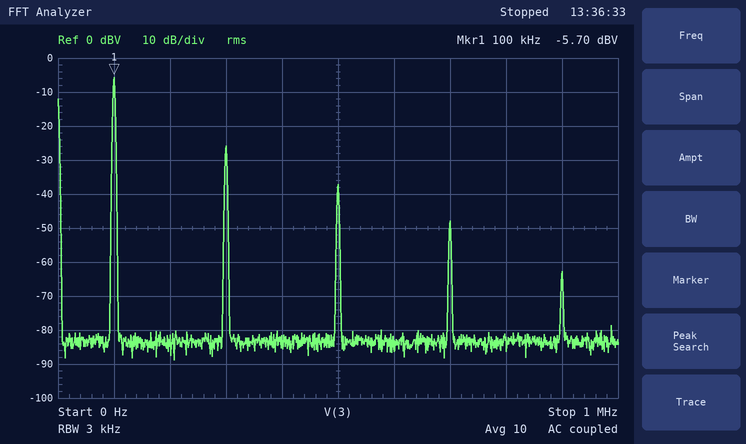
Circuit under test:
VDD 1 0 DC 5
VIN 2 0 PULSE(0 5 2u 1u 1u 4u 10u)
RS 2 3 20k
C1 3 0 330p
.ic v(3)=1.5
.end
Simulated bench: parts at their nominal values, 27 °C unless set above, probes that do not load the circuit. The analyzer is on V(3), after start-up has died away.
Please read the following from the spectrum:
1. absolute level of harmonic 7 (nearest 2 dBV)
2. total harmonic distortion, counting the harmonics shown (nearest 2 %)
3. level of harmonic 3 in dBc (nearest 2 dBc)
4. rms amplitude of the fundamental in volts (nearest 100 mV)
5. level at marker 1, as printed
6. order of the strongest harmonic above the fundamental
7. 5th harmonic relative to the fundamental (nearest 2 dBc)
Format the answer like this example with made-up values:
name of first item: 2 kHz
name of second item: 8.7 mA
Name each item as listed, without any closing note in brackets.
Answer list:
absolute level of harmonic 7: -48 dBV
total harmonic distortion, counting the harmonics shown: 10 %
level of harmonic 3 in dBc: -20 dBc
rms amplitude of the fundamental in volts: 500 mV
level at marker 1, as printed: -5.70 dBV
order of the strongest harmonic above the fundamental: 3
5th harmonic relative to the fundamental: -32 dBc
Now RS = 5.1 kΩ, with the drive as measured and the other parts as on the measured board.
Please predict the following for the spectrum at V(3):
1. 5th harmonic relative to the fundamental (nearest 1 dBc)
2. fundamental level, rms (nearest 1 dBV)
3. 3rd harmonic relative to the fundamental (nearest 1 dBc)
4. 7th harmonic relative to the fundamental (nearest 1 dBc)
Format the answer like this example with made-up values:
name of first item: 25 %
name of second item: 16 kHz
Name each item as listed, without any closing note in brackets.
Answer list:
5th harmonic relative to the fundamental: -29 dBc
fundamental level, rms: 4 dBV
3rd harmonic relative to the fundamental: -18 dBc
7th harmonic relative to the fundamental: -40 dBc
